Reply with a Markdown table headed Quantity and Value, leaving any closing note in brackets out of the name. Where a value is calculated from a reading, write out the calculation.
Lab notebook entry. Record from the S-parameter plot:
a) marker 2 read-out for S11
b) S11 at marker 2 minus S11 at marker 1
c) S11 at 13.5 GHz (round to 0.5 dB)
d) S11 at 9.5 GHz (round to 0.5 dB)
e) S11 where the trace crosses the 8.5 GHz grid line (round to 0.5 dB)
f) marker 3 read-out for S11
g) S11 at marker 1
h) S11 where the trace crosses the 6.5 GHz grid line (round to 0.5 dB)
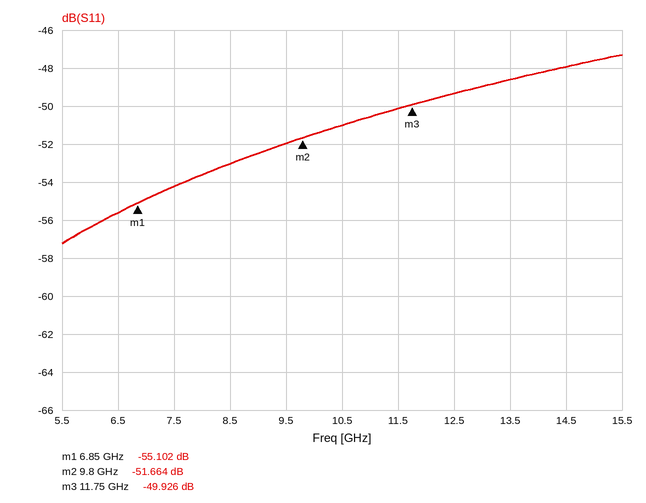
| Quantity | Value |
|---|---|
| marker 2 read-out for S11 | -51.664 dB |
| S11 at marker 2 minus S11 at marker 1 | -51.664 − (-55.102) = 3.438 dB |
| S11 at 13.5 GHz | -48.5 dB |
| S11 at 9.5 GHz | -52.0 dB |
| S11 where the trace crosses the 8.5 GHz grid line | -53.0 dB |
| marker 3 read-out for S11 | -49.926 dB |
| S11 at marker 1 | -55.102 dB |
| S11 where the trace crosses the 6.5 GHz grid line | -55.5 dB |
